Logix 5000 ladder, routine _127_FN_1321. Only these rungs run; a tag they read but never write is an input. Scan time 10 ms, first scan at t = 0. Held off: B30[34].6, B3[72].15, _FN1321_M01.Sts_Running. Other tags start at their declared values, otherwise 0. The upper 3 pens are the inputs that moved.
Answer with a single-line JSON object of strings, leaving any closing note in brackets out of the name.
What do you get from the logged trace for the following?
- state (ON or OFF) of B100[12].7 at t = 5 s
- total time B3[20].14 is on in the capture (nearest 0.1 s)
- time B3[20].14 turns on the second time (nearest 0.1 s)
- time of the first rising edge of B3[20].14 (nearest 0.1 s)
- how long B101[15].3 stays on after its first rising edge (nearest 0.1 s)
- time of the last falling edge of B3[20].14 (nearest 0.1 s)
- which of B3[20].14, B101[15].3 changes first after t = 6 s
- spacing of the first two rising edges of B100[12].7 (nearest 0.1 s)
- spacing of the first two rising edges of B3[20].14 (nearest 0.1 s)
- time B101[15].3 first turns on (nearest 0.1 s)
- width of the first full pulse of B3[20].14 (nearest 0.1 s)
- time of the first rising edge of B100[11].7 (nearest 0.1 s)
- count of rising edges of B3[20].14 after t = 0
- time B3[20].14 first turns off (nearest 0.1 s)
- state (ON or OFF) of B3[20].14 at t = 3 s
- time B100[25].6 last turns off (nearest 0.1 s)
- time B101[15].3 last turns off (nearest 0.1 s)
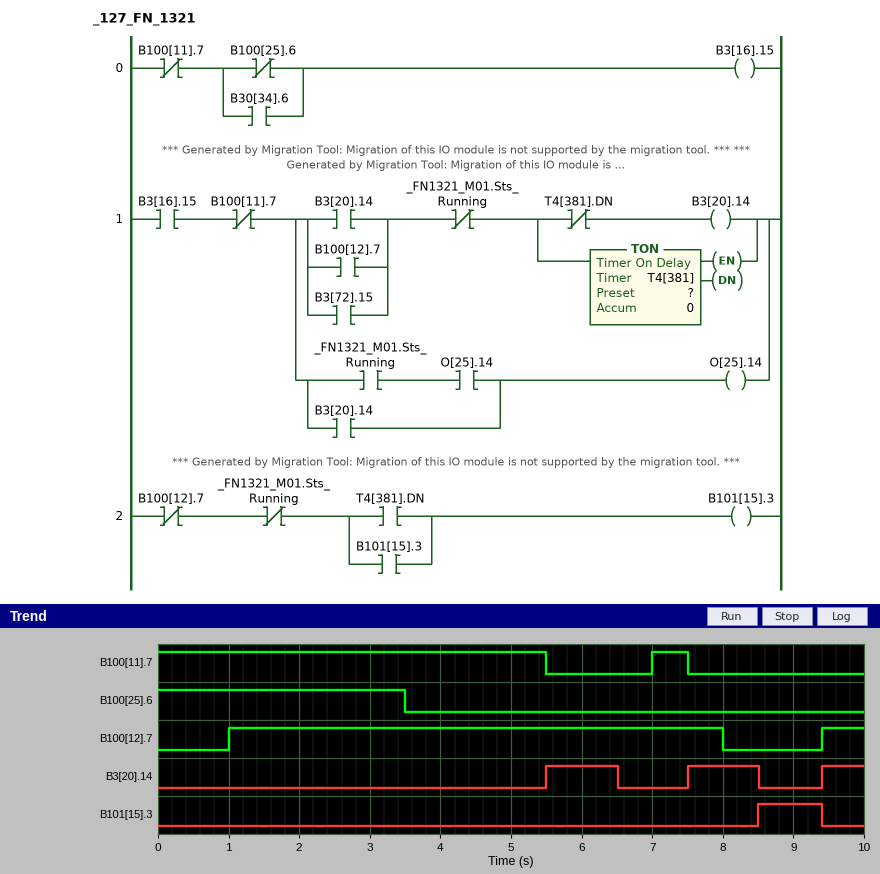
{"state (ON or OFF) of B100[12].7 at t = 5 s": "ON", "total time B3[20].14 is on in the capture": "2.6 s", "time B3[20].14 turns on the second time": "7.5 s", "time of the first rising edge of B3[20].14": "5.5 s", "how long B101[15].3 stays on after its first rising edge": "0.9 s", "time of the last falling edge of B3[20].14": "8.5 s", "which of B3[20].14, B101[15].3 changes first after t = 6 s": "B3[20].14", "spacing of the first two rising edges of B100[12].7": "8.4 s", "spacing of the first two rising edges of B3[20].14": "2.0 s", "time B101[15].3 first turns on": "8.5 s", "width of the first full pulse of B3[20].14": "1.0 s", "time of the first rising edge of B100[11].7": "7.0 s", "count of rising edges of B3[20].14 after t = 0": "3", "time B3[20].14 first turns off": "6.5 s", "state (ON or OFF) of B3[20].14 at t = 3 s": "OFF", "time B100[25].6 last turns off": "3.5 s", "time B101[15].3 last turns off": "9.4 s"}
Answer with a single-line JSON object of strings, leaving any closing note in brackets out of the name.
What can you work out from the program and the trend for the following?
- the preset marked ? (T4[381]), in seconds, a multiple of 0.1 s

{"the preset marked ? (T4[381]), in seconds, a multiple of 0.1 s": "1.0 s"}
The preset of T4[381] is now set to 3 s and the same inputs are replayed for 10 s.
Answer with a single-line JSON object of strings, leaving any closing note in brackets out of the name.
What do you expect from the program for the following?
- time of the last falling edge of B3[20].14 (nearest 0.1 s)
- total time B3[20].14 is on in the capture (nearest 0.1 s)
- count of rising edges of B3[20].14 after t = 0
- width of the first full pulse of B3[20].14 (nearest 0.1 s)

{"time of the last falling edge of B3[20].14": "7.0 s", "total time B3[20].14 is on in the capture": "4.0 s", "count of rising edges of B3[20].14 after t = 0": "2", "width of the first full pulse of B3[20].14": "1.5 s"}
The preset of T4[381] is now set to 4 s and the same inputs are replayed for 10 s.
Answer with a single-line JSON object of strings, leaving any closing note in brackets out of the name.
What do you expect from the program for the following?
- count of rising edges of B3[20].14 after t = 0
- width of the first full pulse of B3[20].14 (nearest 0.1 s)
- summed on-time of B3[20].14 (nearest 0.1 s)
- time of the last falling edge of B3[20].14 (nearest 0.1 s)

{"count of rising edges of B3[20].14 after t = 0": "2", "width of the first full pulse of B3[20].14": "1.5 s", "summed on-time of B3[20].14": "4.0 s", "time of the last falling edge of B3[20].14": "7.0 s"}
